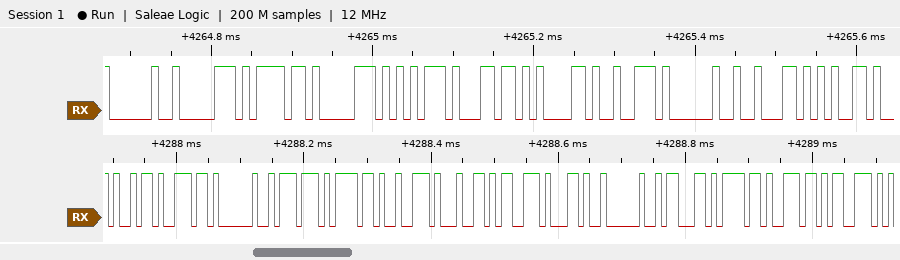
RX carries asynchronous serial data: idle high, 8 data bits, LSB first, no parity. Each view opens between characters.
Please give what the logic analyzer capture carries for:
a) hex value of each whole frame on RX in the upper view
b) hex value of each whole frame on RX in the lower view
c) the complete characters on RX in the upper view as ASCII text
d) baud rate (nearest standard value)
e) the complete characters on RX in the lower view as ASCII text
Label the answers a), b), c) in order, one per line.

a) 20, 70, 6F, 70, 75, 6C, 61, 72, 20, 62, 65
b) 69, 6E, 20, 77, 6F, 72, 64, 73, 2C, 20, 63, 6F, 6E, 73
c) " popular be"
d) 115200 baud
e) "in words, cons"
